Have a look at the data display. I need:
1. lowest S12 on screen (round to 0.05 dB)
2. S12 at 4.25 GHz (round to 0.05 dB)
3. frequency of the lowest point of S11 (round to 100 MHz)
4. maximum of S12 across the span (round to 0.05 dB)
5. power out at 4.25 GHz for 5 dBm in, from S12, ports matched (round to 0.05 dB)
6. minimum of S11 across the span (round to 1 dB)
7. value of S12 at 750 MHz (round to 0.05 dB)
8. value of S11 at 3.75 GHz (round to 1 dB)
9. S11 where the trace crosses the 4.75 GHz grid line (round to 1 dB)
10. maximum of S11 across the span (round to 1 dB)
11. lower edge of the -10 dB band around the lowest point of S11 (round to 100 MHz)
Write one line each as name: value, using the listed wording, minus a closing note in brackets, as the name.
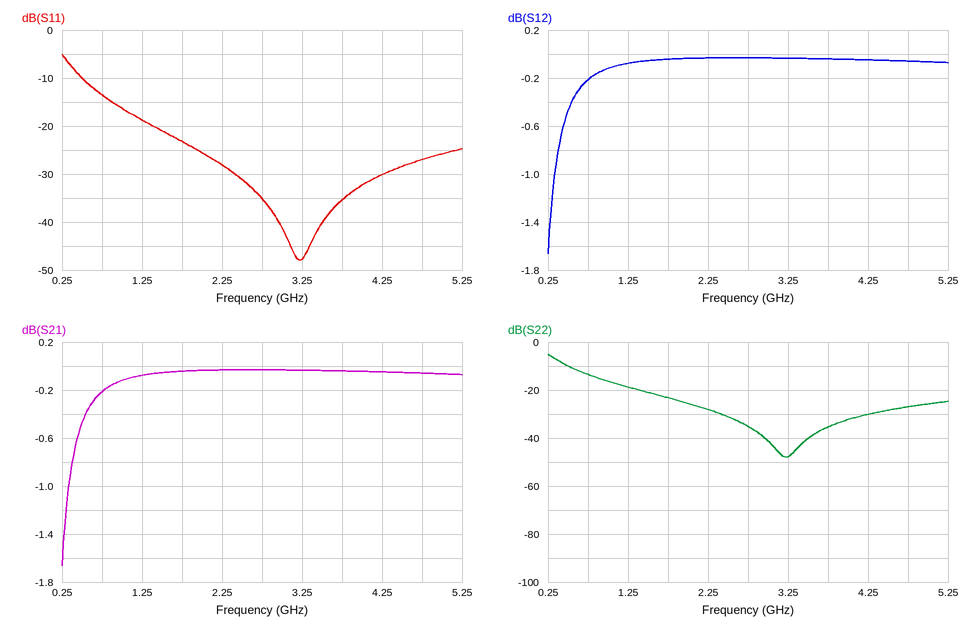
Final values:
lowest S12 on screen: -1.65 dB
S12 at 4.25 GHz: -0.05 dB
frequency of the lowest point of S11: 3.2 GHz
maximum of S12 across the span: -0.05 dB
power out at 4.25 GHz for 5 dBm in, from S12, ports matched: 4.95 dBm
minimum of S11 across the span: -48 dB
value of S12 at 750 MHz: -0.20 dB
value of S11 at 3.75 GHz: -35 dB
S11 where the trace crosses the 4.75 GHz grid line: -27 dB
maximum of S11 across the span: -5 dB
lower edge of the -10 dB band around the lowest point of S11: 500 MHz
